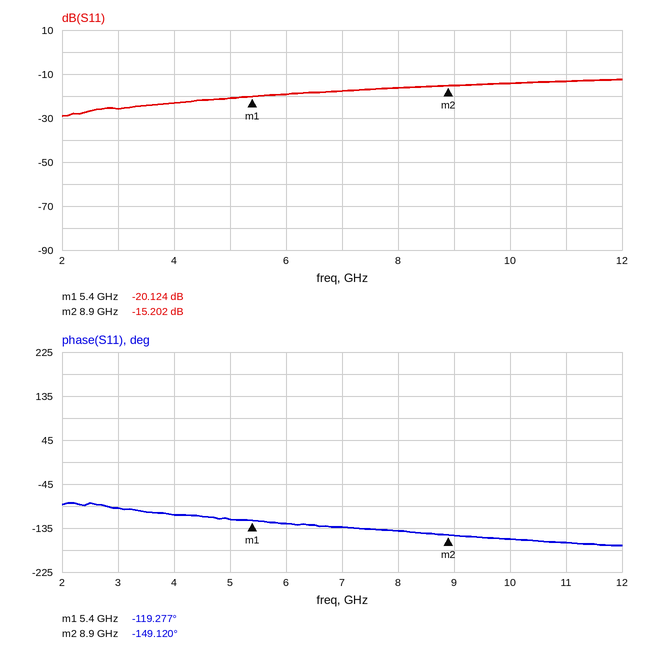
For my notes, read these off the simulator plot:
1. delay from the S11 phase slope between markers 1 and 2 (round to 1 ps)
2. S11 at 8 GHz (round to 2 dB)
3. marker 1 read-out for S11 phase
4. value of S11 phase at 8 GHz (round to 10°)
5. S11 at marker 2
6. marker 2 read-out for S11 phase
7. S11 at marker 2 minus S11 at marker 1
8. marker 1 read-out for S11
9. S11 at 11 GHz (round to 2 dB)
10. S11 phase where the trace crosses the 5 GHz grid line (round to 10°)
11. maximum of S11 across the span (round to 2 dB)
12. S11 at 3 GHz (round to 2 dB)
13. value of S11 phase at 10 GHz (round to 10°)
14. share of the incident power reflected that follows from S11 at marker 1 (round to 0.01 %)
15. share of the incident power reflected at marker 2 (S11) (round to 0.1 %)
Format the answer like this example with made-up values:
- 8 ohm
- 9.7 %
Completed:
- 24 ps
- -16 dB
- -119.277°
- -140°
- -15.202 dB
- -149.120°
- 4.922 dB
- -20.124 dB
- -14 dB
- -120°
- -12 dB
- -26 dB
- -160°
- 0.97 %
- 3.0 %
